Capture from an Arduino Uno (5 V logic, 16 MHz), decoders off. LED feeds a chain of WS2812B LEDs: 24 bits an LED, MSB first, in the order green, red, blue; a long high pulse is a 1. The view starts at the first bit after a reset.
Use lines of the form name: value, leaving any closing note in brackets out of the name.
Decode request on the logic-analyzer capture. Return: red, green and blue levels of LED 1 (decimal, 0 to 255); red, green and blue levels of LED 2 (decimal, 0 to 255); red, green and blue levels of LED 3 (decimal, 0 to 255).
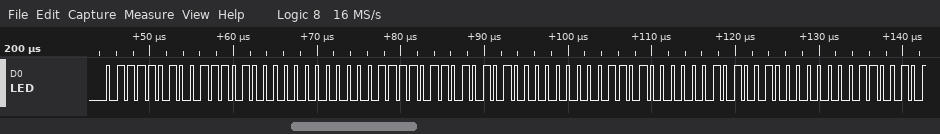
red, green and blue levels of LED 1: 116, 122, 0
red, green and blue levels of LED 2: 170, 61, 0
red, green and blue levels of LED 3: 41, 208, 0
